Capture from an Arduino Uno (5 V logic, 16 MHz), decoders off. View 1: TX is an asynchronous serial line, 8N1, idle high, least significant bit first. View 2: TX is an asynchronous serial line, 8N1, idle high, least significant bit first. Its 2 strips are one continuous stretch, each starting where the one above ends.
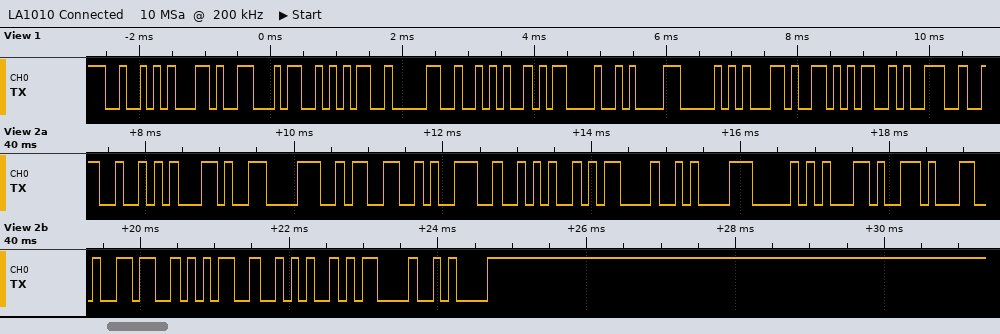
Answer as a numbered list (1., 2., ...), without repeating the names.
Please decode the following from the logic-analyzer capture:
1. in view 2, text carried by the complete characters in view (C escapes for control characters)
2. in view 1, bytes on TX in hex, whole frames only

1. "R,839*\r\nP,165*\r\n"
2. 0x52 0x2C 0x34 0x35 0x30 0x2A 0x0D 0x0A 0x50 0x2C 0x35 0x39
